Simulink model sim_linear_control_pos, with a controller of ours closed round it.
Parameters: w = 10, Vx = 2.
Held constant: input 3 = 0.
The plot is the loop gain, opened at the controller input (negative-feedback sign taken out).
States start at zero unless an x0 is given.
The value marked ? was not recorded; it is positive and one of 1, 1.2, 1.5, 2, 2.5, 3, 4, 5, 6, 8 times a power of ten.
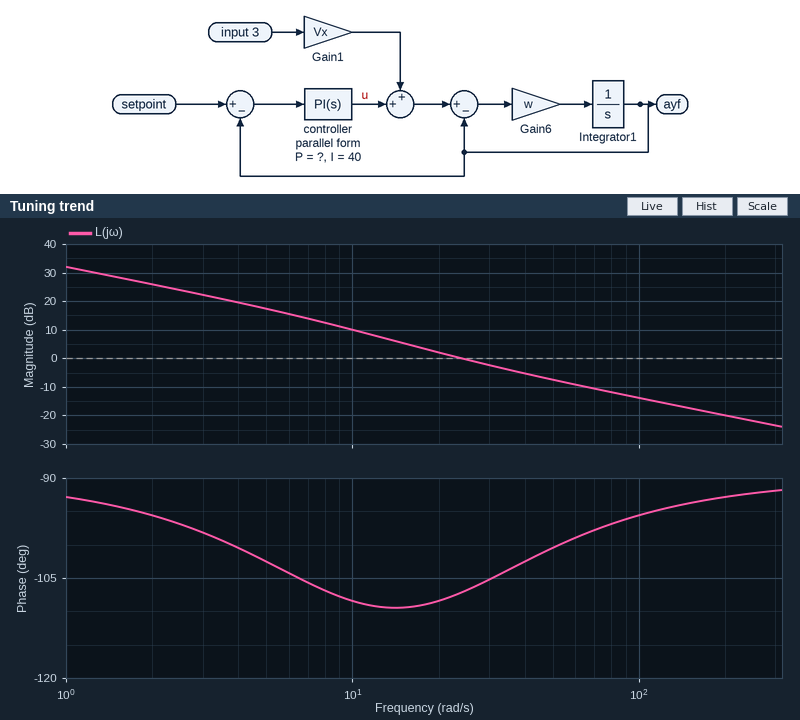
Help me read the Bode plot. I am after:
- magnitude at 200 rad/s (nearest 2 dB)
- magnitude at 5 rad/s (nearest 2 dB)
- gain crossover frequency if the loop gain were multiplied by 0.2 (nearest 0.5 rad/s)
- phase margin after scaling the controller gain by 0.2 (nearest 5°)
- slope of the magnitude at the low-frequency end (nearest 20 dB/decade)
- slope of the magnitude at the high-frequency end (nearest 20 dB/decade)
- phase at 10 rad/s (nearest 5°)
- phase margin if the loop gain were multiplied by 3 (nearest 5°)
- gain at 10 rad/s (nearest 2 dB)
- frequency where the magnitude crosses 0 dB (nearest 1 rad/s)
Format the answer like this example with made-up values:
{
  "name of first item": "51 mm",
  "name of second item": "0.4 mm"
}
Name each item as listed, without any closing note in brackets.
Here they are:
{
  "magnitude at 200 rad/s": "-20 dB",
  "magnitude at 5 rad/s": "18 dB",
  "gain crossover frequency if the loop gain were multiplied by 0.2": "7.0 rad/s",
  "phase margin after scaling the controller gain by 0.2": "75°",
  "slope of the magnitude at the low-frequency end": "-20 dB/decade",
  "slope of the magnitude at the high-frequency end": "-20 dB/decade",
  "phase at 10 rad/s": "-110°",
  "phase margin if the loop gain were multiplied by 3": "80°",
  "gain at 10 rad/s": "10 dB",
  "frequency where the magnitude crosses 0 dB": "24 rad/s"
}
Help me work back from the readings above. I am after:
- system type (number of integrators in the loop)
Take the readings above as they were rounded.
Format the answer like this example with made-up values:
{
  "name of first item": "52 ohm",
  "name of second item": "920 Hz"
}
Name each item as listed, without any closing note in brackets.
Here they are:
{
  "system type": "1"
}
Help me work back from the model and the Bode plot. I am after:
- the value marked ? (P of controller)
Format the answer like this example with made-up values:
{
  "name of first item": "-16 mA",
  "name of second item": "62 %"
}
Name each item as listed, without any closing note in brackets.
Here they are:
{
  "the value marked ?": "2"
}
